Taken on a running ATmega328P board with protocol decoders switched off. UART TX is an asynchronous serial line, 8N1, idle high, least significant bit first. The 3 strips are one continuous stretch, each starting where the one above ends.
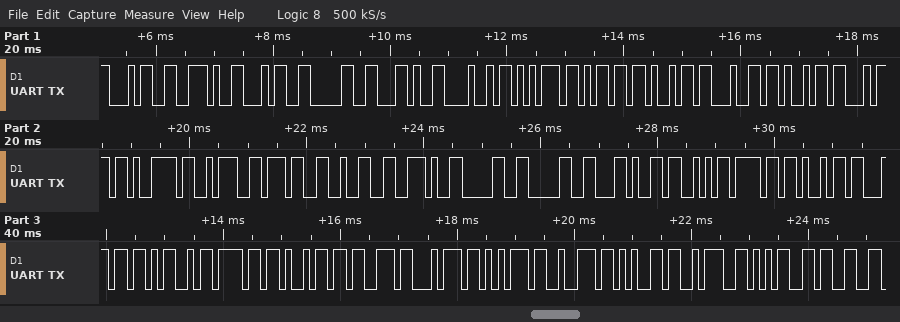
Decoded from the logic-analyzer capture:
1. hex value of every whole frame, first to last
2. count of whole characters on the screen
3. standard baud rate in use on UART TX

34 2E 34 30 2C 48 75 6D 69 64 69 74 79 3A 37 32 2E 30 30 2C 53 6F 69 6C 4D 6F 69 73 74 75 72 65 3A 35 33
35
9600 baud
